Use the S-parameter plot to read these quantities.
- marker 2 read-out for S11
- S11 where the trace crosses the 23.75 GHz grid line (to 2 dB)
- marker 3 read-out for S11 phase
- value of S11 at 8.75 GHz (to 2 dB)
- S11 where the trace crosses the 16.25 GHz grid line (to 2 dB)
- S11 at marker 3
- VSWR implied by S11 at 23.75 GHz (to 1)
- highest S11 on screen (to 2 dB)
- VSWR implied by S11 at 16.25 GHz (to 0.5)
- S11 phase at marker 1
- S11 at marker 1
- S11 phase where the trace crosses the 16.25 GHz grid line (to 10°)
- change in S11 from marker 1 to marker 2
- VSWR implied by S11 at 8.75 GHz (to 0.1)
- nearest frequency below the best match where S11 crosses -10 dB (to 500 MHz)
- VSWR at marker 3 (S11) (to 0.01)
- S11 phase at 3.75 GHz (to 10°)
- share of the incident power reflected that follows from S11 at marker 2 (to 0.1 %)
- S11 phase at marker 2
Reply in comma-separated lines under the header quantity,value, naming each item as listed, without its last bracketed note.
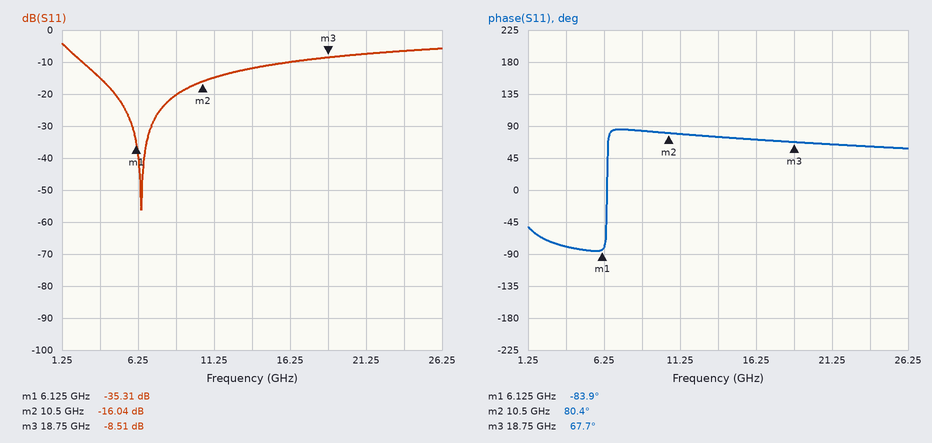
quantity,value
marker 2 read-out for S11,-16.04 dB
S11 where the trace crosses the 23.75 GHz grid line,-6 dB
marker 3 read-out for S11 phase,67.7°
value of S11 at 8.75 GHz,-20 dB
S11 where the trace crosses the 16.25 GHz grid line,-10 dB
S11 at marker 3,-8.51 dB
VSWR implied by S11 at 23.75 GHz,3
highest S11 on screen,-4 dB
VSWR implied by S11 at 16.25 GHz,2.0
S11 phase at marker 1,-83.9°
S11 at marker 1,-35.31 dB
S11 phase where the trace crosses the 16.25 GHz grid line,70°
change in S11 from marker 1 to marker 2,19.27 dB
VSWR implied by S11 at 8.75 GHz,1.2
nearest frequency below the best match where S11 crosses -10 dB,2.5 GHz
VSWR at marker 3 (S11),2.20
S11 phase at 3.75 GHz,-80°
share of the incident power reflected that follows from S11 at marker 2,2.5 %
S11 phase at marker 2,80.4°
